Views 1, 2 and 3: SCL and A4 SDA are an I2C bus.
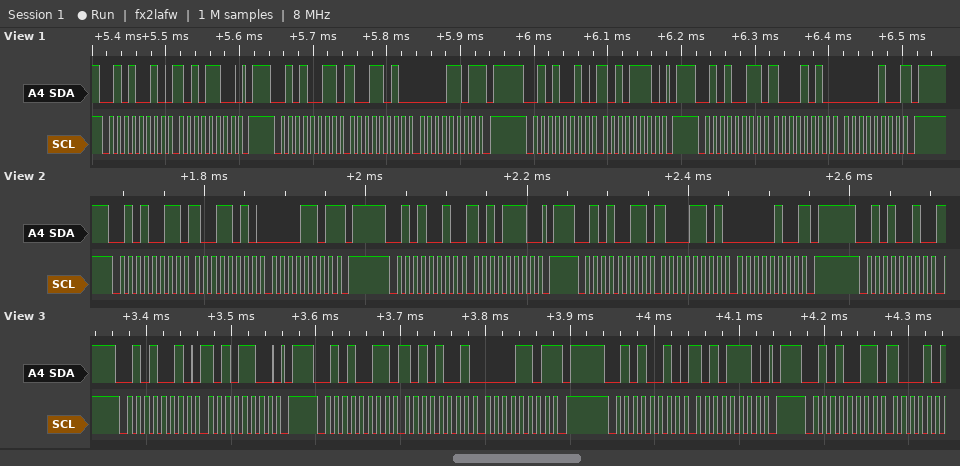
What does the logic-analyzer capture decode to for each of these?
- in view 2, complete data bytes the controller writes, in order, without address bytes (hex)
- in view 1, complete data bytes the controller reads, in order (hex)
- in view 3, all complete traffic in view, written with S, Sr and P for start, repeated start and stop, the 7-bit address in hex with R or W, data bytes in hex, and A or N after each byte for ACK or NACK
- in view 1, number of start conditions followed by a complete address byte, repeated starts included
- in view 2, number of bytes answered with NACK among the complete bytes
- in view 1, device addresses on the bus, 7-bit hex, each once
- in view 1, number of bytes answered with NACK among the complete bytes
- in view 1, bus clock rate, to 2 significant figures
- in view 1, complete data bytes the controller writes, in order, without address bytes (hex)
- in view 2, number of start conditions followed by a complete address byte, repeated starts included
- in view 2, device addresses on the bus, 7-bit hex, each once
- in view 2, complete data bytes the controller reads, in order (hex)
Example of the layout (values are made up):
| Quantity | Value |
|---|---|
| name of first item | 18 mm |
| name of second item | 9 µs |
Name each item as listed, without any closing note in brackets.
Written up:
| Quantity | Value |
|---|---|
| in view 2, complete data bytes the controller writes, in order, without address bytes | AE |
| in view 1, complete data bytes the controller reads, in order | 9A 0D 8A 04 |
| in view 3, all complete traffic in view, written with S, Sr and P for start, repeated start and stop, the 7-bit address in hex with R or W, data bytes in hex, and A or N after each byte for ACK or NACK | S 29W A AC A P S 29R A A9 A 0D N P S 29W A AE A P S 29R A |
| in view 1, number of start conditions followed by a complete address byte, repeated starts included | 4 |
| in view 2, number of bytes answered with NACK among the complete bytes | 2 |
| in view 1, device addresses on the bus, 7-bit hex, each once | 0x29 |
| in view 1, number of bytes answered with NACK among the complete bytes | 2 |
| in view 1, bus clock rate, to 2 significant figures | 100 kHz |
| in view 1, complete data bytes the controller writes, in order, without address bytes | AC AE |
| in view 2, number of start conditions followed by a complete address byte, repeated starts included | 4 |
| in view 2, device addresses on the bus, 7-bit hex, each once | 0x29 |
| in view 2, complete data bytes the controller reads, in order | 9A 0D 8D 04 |
